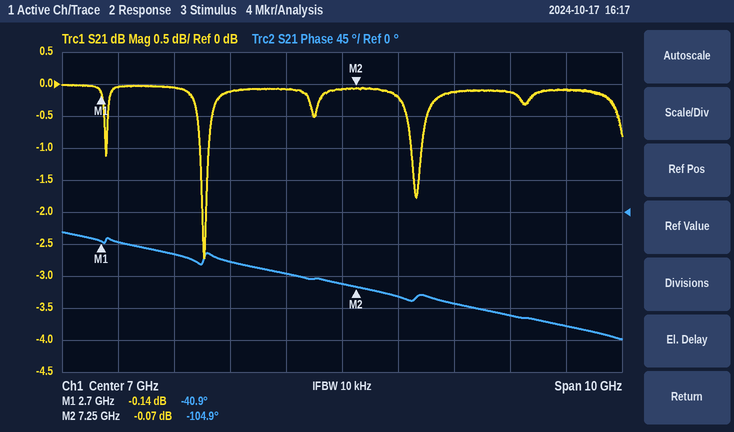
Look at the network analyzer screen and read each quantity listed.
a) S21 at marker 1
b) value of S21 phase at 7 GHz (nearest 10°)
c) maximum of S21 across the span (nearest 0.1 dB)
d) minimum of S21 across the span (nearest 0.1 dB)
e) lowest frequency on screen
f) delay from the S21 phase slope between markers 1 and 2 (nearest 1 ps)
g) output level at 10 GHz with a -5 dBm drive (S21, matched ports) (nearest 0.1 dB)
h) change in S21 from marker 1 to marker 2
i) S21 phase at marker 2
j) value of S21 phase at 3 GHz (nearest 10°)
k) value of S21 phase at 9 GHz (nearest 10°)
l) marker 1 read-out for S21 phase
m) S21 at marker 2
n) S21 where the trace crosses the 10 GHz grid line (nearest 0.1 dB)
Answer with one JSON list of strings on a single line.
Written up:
["-0.14 dB", "-100°", "0.0 dB", "-2.7 dB", "2 GHz", "39 ps", "-5.1 dBm", "0.07 dB", "-104.9°", "-40°", "-130°", "-40.9°", "-0.07 dB", "-0.1 dB"]
